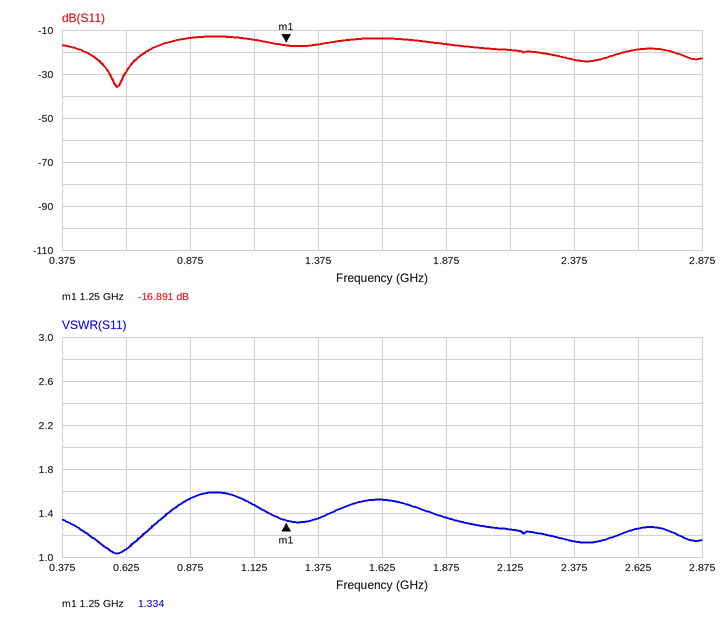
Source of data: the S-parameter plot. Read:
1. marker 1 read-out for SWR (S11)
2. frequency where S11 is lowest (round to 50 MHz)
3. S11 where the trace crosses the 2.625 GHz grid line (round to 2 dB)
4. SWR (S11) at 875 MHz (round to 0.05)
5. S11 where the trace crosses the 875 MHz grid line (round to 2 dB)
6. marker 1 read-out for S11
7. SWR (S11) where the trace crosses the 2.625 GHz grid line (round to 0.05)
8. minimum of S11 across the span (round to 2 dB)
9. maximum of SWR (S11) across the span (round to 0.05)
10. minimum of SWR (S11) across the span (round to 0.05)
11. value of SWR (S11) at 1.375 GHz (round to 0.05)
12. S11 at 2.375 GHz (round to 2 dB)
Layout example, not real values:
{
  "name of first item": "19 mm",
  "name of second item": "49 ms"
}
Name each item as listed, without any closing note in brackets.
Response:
{
  "marker 1 read-out for SWR": "1.334",
  "frequency where S11 is lowest": "600 MHz",
  "S11 where the trace crosses the 2.625 GHz grid line": "-18 dB",
  "SWR (S11) at 875 MHz": "1.55",
  "S11 where the trace crosses the 875 MHz grid line": "-14 dB",
  "marker 1 read-out for S11": "-16.891 dB",
  "SWR (S11) where the trace crosses the 2.625 GHz grid line": "1.25",
  "minimum of S11 across the span": "-36 dB",
  "maximum of SWR (S11) across the span": "1.60",
  "minimum of SWR (S11) across the span": "1.05",
  "value of SWR (S11) at 1.375 GHz": "1.35",
  "S11 at 2.375 GHz": "-24 dB"
}
